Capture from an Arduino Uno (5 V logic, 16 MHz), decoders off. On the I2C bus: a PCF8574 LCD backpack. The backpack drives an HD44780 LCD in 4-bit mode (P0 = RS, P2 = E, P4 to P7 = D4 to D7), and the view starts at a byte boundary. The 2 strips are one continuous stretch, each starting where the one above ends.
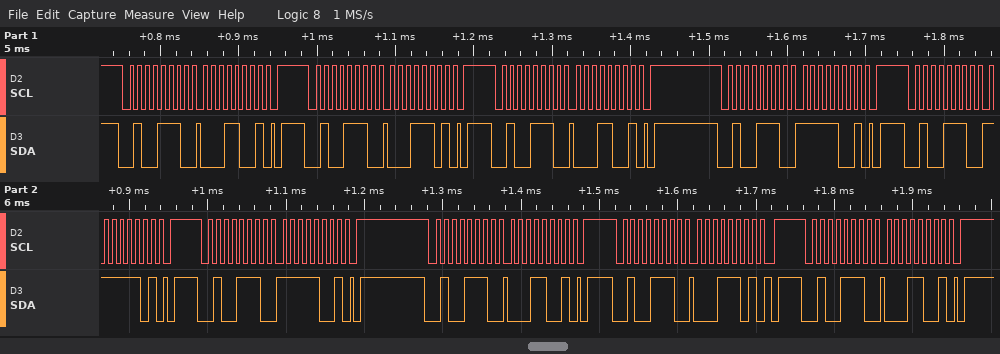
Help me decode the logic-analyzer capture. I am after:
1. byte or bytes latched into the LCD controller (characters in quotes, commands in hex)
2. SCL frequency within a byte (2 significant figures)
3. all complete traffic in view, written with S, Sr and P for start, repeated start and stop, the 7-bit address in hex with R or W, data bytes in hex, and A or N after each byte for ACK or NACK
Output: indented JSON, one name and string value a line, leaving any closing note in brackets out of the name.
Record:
{
  "byte or bytes latched into the LCD controller": "data 0x1F",
  "SCL frequency within a byte": "100 kHz",
  "all complete traffic in view, written with S, Sr and P for start, repeated start and stop, the 7-bit address in hex with R or W, data bytes in hex, and A or N after each byte for ACK or NACK": "S 27W A 19 A P S 27W A 1D A P S 27W A 19 A P S 27W A F9 A P S 27W A FD A P S 27W A F9 A P S 27W A 19 A P S 27W A 1D A P S 27W A 19 A P"
}
